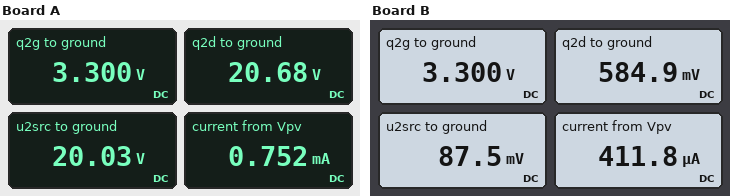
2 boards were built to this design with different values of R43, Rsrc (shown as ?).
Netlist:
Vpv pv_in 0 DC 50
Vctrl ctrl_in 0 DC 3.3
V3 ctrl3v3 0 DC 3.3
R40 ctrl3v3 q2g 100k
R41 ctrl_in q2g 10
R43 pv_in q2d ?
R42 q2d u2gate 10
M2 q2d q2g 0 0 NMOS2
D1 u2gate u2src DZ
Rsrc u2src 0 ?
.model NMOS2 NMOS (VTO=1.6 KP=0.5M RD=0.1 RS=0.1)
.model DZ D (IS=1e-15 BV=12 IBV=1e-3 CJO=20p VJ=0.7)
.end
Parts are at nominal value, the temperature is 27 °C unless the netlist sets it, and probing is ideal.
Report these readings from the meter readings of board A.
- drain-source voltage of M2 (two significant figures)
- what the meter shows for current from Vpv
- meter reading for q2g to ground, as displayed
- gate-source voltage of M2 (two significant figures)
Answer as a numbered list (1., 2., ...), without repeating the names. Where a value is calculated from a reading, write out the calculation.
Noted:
1. 20.68 V = 21 V
2. 0.752 mA
3. 3.300 V
4. 3.3 V = 3.3 V
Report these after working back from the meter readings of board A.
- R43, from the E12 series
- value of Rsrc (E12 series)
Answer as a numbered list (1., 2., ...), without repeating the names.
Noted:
1. 39 kΩ
2. 680 kΩ
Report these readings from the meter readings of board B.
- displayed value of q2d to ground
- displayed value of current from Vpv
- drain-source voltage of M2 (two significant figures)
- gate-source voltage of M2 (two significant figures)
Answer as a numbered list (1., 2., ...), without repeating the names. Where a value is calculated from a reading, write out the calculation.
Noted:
1. 584.9 mV
2. 411.8 µA
3. 584.9 mV = 580 mV
4. 3.3 V = 3.3 V
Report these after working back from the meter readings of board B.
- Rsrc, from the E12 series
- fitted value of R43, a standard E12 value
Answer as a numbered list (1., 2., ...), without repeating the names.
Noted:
1. 390 kΩ
2. 120 kΩ
